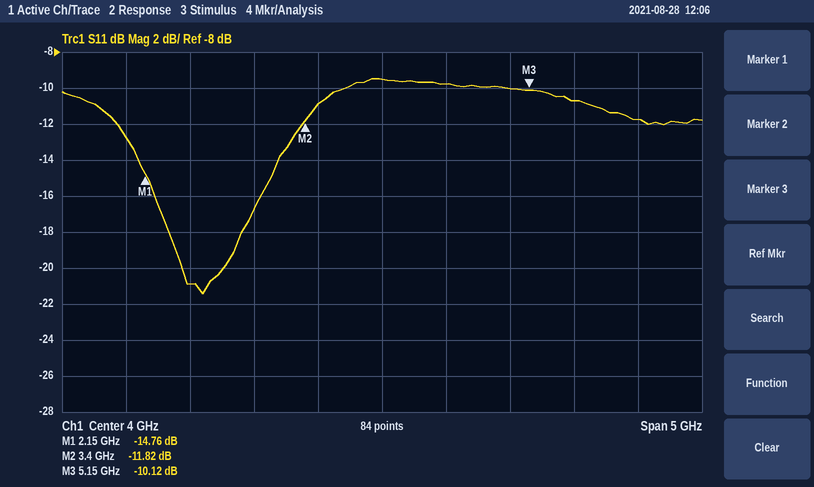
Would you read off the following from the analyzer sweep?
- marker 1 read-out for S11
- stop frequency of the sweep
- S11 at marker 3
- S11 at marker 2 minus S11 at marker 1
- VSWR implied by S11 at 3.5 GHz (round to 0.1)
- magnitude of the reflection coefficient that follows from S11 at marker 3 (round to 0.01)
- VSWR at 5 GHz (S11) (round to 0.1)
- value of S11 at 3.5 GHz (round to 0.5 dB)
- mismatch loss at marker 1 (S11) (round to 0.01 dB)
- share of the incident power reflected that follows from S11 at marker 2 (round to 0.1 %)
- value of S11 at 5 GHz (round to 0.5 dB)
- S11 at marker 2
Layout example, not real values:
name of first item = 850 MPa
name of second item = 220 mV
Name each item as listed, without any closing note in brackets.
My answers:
marker 1 read-out for S11 = -14.76 dB
stop frequency of the sweep = 6.5 GHz
S11 at marker 3 = -10.12 dB
S11 at marker 2 minus S11 at marker 1 = 2.94 dB
VSWR implied by S11 at 3.5 GHz = 1.8
magnitude of the reflection coefficient that follows from S11 at marker 3 = 0.31
VSWR at 5 GHz (S11) = 1.9
value of S11 at 3.5 GHz = -11.0 dB
mismatch loss at marker 1 (S11) = 0.15 dB
share of the incident power reflected that follows from S11 at marker 2 = 6.6 %
value of S11 at 5 GHz = -10.0 dB
S11 at marker 2 = -11.82 dB
